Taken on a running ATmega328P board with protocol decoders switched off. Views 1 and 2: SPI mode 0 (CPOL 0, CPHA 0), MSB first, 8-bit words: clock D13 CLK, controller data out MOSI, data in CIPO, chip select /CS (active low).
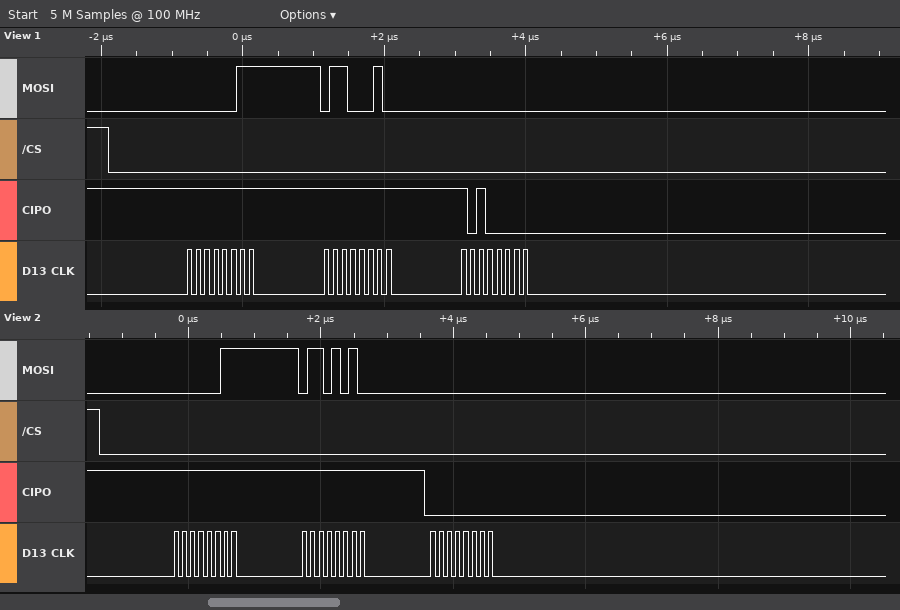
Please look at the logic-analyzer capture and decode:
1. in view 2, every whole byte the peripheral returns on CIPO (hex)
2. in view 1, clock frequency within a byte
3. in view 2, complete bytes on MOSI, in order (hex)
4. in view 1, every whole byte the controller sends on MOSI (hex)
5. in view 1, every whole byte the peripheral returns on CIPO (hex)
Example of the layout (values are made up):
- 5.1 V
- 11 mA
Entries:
- FF FF 00
- 8 MHz
- 03 6A 00
- 0x03 0x62 0x00
- 0xFF 0xFF 0xA0
